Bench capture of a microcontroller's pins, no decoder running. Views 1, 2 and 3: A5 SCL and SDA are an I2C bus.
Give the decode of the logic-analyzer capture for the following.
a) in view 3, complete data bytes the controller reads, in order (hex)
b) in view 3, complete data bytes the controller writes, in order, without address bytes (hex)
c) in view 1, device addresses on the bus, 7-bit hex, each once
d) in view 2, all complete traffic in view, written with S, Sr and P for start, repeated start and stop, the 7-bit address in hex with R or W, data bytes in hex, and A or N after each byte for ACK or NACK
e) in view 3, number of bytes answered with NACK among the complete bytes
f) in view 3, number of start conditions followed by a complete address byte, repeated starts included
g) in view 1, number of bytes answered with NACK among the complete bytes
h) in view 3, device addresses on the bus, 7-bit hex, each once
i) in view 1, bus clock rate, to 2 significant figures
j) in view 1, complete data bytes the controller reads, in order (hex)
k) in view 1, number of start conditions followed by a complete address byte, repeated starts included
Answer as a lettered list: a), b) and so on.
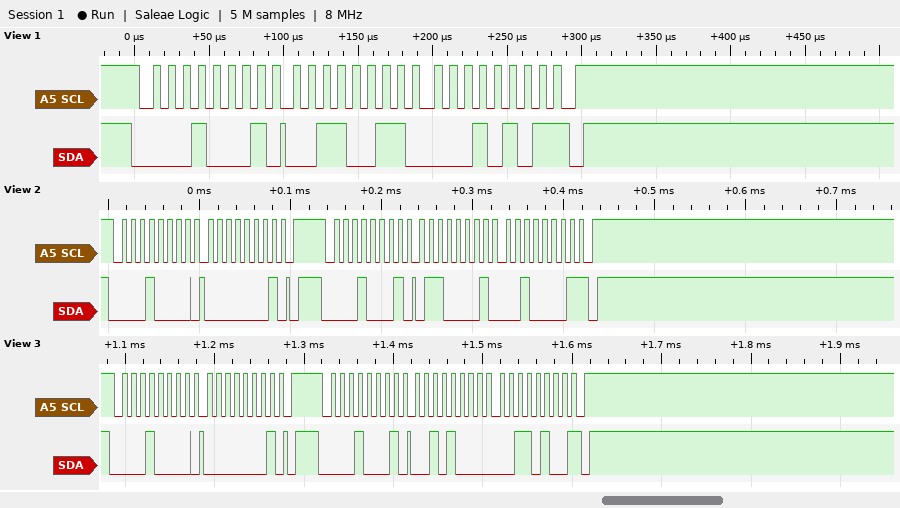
a) 28 34
b) 01
c) 0x08
d) S 08W A 01 A P S 08R A 61 A 21 N P
e) 1
f) 2
g) 1
h) 0x08
i) 100 kHz
j) 33 15
k) 1
